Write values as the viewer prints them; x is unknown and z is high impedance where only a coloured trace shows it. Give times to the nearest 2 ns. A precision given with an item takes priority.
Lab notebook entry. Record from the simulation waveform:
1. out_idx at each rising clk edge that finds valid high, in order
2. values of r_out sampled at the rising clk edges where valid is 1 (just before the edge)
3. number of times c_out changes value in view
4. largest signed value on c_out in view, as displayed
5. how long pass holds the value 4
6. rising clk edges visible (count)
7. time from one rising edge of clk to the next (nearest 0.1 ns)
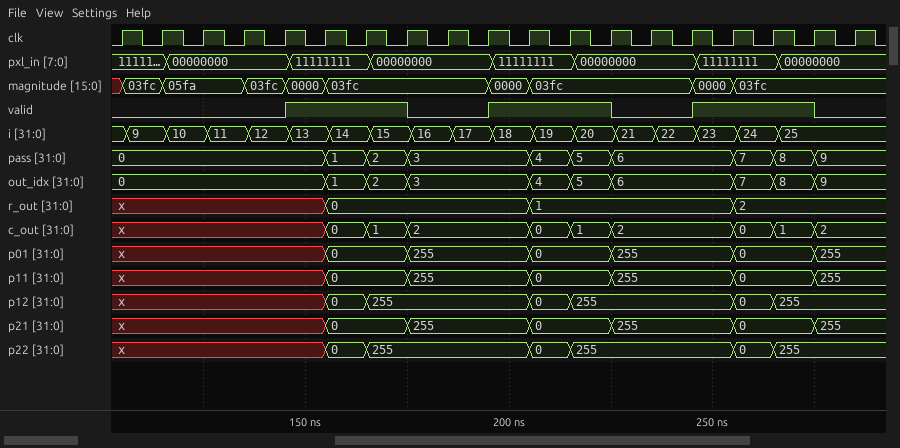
0, 1, 2, 3, 4, 5, 6, 7, 8
x, 0, 0, 0, 1, 1, 1, 2, 2
9
2
10 ns
19
10 ns
